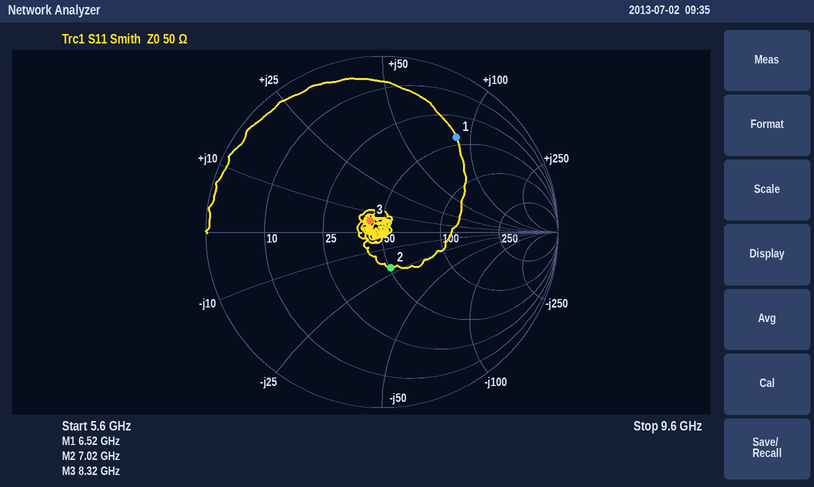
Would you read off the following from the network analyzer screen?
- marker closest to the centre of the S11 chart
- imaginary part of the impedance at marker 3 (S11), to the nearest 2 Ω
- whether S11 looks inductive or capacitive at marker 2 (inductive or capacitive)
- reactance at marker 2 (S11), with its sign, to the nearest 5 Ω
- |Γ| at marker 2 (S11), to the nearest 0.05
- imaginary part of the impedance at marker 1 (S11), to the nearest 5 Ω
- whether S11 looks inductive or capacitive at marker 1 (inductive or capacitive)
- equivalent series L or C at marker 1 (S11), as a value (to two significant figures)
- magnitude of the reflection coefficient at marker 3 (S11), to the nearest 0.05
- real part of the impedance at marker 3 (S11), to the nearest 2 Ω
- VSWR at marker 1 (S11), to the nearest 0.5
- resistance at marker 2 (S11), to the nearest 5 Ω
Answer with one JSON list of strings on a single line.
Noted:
["marker 3", "+6 Ω", "capacitive", "-20 Ω", "0.20", "+85 Ω", "inductive", "2.1 nH", "0.10", "44 Ω", "5.5", "50 Ω"]
